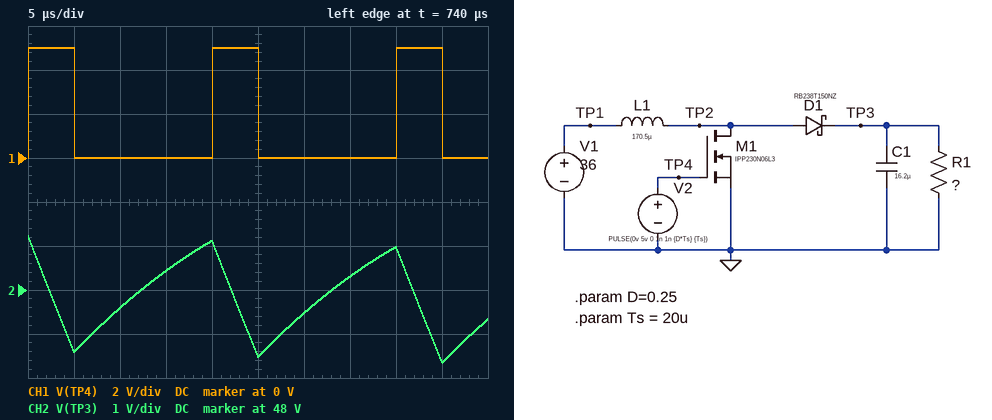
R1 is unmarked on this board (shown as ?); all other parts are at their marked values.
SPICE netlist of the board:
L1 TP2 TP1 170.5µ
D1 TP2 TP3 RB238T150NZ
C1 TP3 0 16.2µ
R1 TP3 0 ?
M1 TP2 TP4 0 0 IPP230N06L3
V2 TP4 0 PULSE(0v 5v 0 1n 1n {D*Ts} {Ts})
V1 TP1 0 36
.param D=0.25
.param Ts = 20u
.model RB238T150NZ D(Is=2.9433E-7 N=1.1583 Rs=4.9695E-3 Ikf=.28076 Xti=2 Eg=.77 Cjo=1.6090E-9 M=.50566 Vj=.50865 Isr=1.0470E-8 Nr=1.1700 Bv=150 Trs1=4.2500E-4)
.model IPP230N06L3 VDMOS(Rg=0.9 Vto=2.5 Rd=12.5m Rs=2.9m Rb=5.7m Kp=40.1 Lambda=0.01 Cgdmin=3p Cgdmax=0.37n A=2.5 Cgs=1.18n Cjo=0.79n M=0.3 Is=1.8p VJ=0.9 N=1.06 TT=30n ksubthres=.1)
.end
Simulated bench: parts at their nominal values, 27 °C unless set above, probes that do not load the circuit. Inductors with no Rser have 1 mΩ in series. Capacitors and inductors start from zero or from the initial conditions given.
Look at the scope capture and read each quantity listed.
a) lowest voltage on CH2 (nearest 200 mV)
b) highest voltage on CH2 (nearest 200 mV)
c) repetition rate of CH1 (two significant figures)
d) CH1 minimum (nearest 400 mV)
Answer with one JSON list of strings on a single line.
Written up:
["46.4 V", "49.2 V", "50 kHz", "0 V"]
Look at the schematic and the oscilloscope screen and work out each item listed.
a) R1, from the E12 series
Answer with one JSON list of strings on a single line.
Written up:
["5.6 Ω"]
